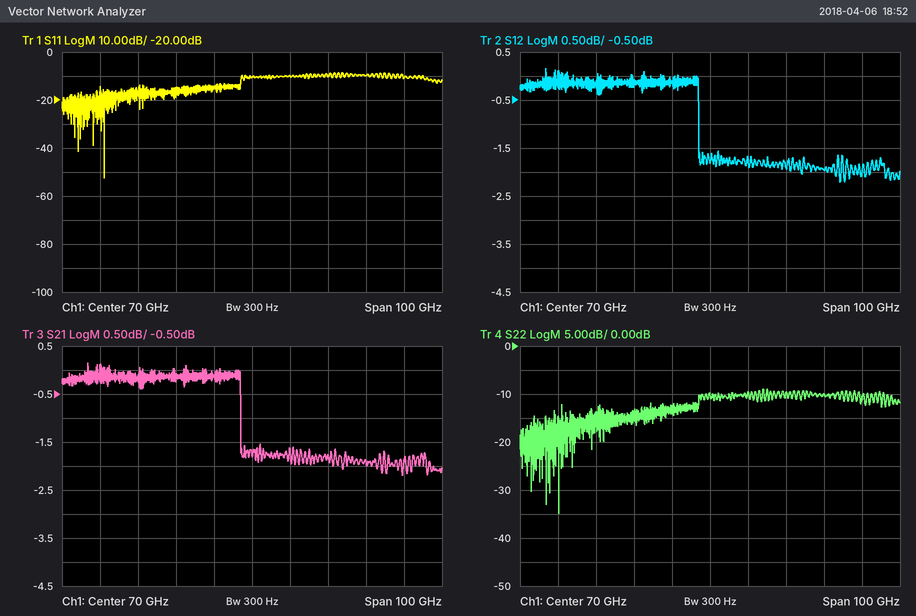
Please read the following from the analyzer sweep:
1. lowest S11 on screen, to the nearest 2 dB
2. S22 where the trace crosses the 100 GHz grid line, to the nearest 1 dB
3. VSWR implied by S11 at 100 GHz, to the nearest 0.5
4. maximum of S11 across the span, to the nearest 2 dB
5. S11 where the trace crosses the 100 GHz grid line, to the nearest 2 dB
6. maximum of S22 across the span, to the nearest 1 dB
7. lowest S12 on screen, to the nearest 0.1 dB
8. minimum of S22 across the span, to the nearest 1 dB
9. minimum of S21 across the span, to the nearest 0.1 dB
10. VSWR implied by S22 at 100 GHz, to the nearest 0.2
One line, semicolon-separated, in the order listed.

-52 dB; -10 dB; 2.0; -8 dB; -10 dB; -9 dB; -2.2 dB; -35 dB; -2.2 dB; 2.0
